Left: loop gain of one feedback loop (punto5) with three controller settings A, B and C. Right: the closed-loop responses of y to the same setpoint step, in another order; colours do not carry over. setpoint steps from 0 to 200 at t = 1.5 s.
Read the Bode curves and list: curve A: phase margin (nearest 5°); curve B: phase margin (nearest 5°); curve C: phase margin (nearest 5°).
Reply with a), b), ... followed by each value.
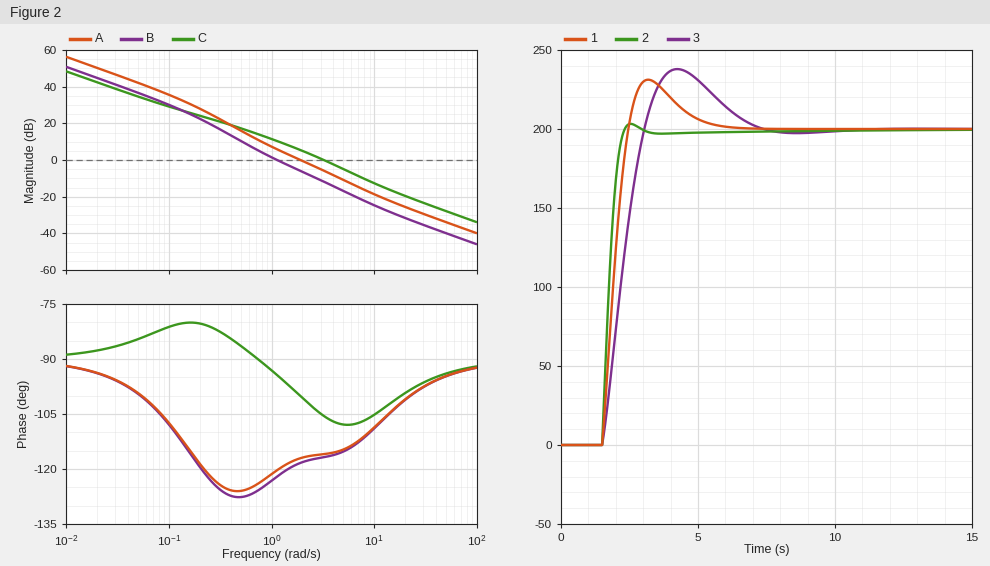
a) 65°
b) 60°
c) 75°
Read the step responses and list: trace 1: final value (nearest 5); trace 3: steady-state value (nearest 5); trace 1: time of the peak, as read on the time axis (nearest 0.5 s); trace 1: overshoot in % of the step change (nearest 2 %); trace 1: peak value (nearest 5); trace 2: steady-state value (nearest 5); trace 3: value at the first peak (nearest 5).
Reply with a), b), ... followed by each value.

a) 200
b) 200
c) 3.0 s
d) 16 %
e) 230
f) 200
g) 240
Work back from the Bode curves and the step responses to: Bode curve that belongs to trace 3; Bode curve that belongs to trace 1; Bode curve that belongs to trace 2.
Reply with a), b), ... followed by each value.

a) B
b) A
c) C
